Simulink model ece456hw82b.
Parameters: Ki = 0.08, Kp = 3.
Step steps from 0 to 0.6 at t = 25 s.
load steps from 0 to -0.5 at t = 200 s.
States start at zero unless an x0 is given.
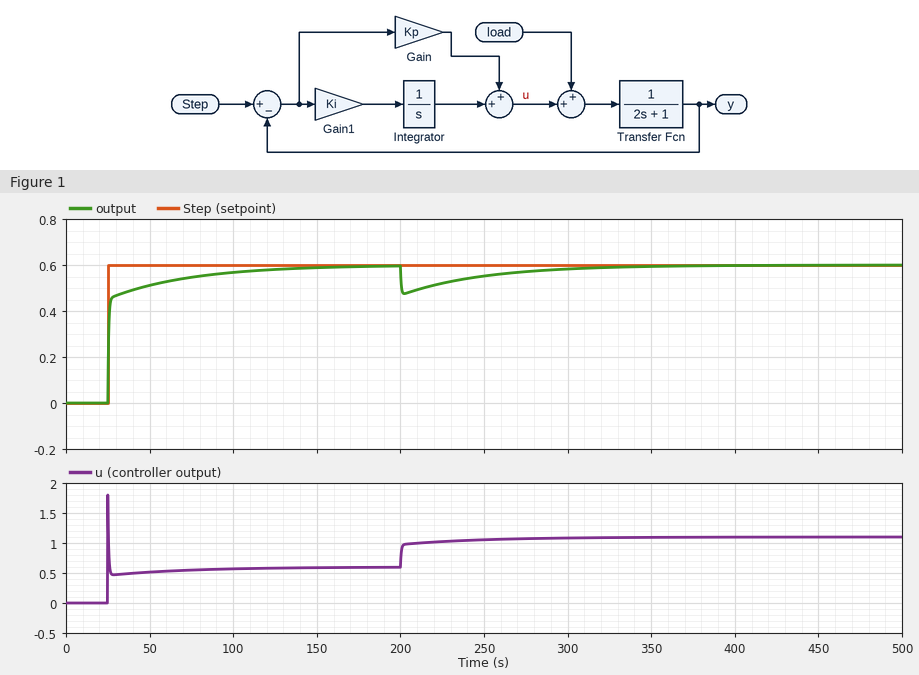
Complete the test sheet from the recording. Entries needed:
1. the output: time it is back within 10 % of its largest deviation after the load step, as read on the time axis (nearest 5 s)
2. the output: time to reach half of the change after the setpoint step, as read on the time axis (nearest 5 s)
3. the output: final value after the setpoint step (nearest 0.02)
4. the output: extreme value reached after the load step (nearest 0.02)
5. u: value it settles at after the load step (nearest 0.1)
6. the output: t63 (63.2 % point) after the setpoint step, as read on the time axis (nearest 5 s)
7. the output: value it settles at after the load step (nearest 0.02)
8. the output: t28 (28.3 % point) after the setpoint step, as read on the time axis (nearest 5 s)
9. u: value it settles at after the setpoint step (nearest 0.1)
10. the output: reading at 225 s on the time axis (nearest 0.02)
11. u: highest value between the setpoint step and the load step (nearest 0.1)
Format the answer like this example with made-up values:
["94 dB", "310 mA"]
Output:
["320 s", "25 s", "0.60", "0.48", "1.1", "25 s", "0.60", "25 s", "0.6", "0.52", "1.8"]
